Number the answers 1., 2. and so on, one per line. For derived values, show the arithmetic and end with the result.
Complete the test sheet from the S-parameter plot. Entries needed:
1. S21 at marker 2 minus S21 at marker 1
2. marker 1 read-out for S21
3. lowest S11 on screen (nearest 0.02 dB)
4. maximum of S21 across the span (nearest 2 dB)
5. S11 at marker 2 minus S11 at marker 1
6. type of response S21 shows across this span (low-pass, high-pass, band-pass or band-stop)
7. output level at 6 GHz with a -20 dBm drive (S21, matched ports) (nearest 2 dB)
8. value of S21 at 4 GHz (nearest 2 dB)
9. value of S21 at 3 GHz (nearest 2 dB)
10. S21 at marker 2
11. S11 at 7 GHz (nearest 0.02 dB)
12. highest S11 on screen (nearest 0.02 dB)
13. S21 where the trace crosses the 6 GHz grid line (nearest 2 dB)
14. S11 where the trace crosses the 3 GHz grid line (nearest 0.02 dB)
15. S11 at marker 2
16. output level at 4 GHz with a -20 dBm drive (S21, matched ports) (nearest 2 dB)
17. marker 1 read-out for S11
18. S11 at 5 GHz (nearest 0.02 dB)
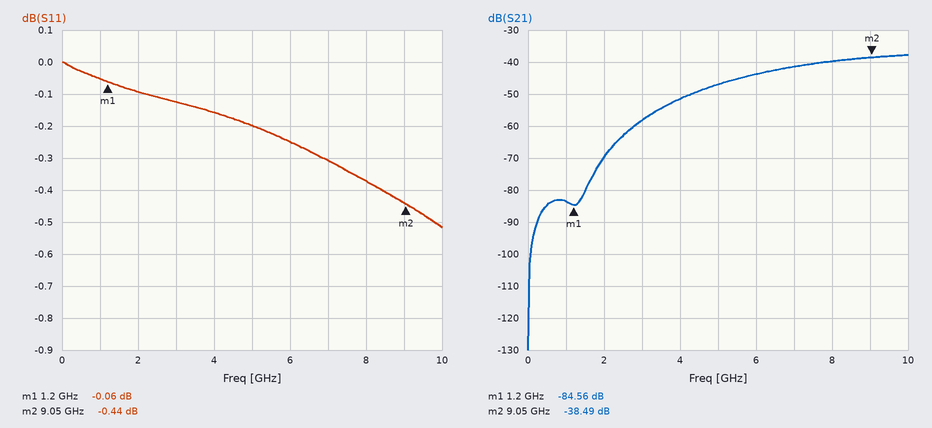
1. -38.49 − (-84.56) = 46.07 dB
2. -84.56 dB
3. -0.52 dB
4. -38 dB
5. -0.44 − (-0.06) = -0.38 dB
6. high-pass
7. -20 dBm + (-44 dB) = -64 dBm
8. -52 dB
9. -58 dB
10. -38.49 dB
11. -0.30 dB
12. 0.00 dB
13. -44 dB
14. -0.12 dB
15. -0.44 dB
16. -20 dBm + (-52 dB) = -72 dBm
17. -0.06 dB
18. -0.20 dB
